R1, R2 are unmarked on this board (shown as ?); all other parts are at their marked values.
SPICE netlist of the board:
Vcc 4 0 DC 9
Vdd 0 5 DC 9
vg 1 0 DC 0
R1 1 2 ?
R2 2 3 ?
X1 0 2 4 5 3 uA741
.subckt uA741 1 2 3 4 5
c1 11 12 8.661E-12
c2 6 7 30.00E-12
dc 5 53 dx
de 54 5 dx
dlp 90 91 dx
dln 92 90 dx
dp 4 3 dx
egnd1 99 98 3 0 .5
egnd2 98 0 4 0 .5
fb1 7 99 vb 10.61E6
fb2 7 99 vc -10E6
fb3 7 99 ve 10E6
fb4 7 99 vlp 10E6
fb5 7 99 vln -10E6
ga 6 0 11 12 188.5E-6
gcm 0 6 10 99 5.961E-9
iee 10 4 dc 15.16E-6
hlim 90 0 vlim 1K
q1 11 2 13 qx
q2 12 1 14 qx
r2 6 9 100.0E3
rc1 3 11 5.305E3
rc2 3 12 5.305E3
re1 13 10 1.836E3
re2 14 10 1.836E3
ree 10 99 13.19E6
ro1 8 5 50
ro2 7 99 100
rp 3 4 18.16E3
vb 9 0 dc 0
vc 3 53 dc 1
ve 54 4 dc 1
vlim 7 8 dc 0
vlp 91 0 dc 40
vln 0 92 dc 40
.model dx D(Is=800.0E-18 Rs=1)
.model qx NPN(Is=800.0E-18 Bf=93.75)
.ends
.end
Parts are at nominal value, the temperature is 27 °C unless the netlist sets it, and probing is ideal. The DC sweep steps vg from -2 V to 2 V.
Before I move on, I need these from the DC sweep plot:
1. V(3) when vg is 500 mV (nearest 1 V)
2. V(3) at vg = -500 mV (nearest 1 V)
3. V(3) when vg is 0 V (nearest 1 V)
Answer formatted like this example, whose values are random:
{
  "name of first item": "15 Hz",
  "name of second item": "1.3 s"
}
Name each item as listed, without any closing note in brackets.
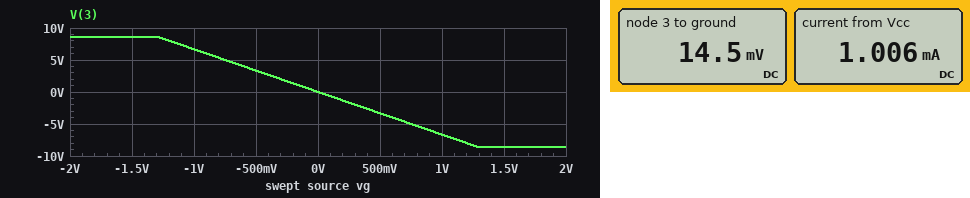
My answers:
{
  "V(3) when vg is 500 mV": "-3 V",
  "V(3) at vg = -500 mV": "3 V",
  "V(3) when vg is 0 V": "0 V"
}
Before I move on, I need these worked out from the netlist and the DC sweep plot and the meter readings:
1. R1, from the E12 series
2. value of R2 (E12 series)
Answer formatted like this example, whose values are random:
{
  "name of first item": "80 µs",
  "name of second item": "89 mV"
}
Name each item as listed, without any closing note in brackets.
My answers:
{
  "R1, from the E12 series": "27 kΩ",
  "value of R2": "180 kΩ"
}
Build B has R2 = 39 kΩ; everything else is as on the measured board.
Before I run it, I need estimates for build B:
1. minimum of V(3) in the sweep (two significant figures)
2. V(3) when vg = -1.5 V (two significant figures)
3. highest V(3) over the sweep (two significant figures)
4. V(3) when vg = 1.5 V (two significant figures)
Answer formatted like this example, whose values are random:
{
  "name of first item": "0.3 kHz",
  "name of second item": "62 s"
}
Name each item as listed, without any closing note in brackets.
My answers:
{
  "minimum of V(3) in the sweep": "-2.9 V",
  "V(3) when vg = -1.5 V": "2.2 V",
  "highest V(3) over the sweep": "2.9 V",
  "V(3) when vg = 1.5 V": "-2.2 V"
}
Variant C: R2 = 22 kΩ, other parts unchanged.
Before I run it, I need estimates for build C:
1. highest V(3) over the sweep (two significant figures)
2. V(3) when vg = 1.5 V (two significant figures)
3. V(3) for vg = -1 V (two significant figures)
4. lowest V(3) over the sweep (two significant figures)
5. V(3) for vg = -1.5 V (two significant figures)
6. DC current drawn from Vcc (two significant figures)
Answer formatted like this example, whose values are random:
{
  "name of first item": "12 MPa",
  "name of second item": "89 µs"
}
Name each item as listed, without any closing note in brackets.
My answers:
{
  "highest V(3) over the sweep": "1.6 V",
  "V(3) when vg = 1.5 V": "-1.2 V",
  "V(3) for vg = -1 V": "820 mV",
  "lowest V(3) over the sweep": "-1.6 V",
  "V(3) for vg = -1.5 V": "1.2 V",
  "DC current drawn from Vcc": "1.0 mA"
}
